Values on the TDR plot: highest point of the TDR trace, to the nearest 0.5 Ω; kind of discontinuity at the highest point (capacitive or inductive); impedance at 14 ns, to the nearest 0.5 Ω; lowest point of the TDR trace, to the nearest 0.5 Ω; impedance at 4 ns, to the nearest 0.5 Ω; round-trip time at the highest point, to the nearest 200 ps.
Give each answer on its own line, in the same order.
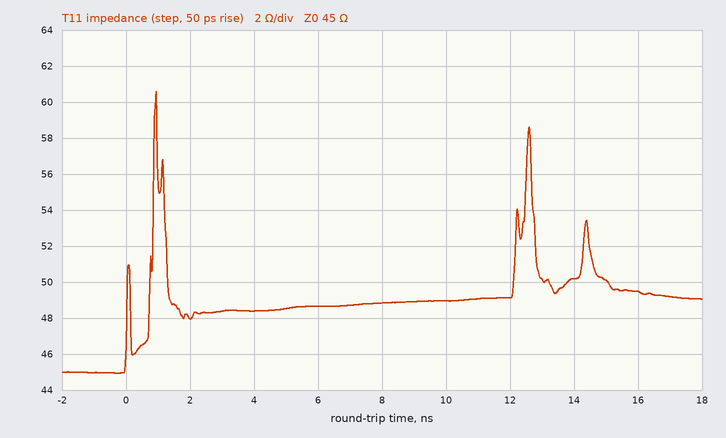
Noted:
60.5 Ω
inductive
50.0 Ω
45.0 Ω
48.5 Ω
1.0 ns
